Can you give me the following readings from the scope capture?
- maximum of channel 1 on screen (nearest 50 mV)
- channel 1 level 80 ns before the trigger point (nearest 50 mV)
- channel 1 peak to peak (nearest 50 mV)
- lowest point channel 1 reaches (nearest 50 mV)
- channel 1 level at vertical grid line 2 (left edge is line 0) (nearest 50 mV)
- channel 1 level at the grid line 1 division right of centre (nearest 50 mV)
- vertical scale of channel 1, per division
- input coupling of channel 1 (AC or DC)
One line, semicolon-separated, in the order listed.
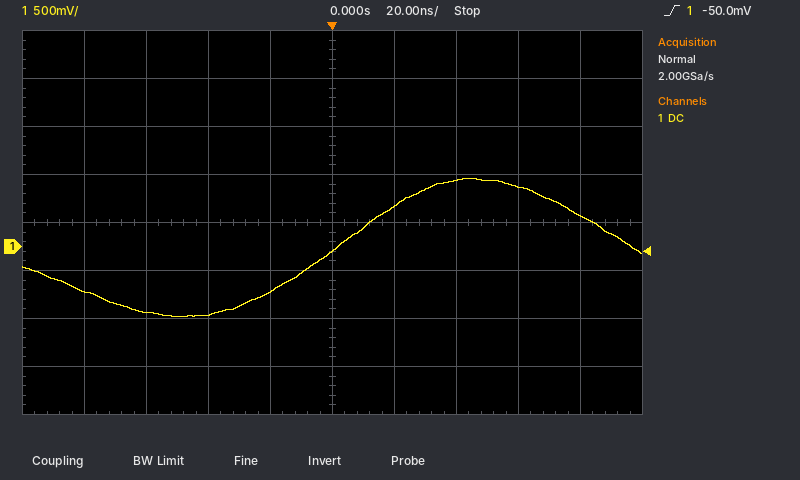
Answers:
700 mV; -450 mV; 1.45 V; -750 mV; -700 mV; 400 mV; 500 mV; DC
